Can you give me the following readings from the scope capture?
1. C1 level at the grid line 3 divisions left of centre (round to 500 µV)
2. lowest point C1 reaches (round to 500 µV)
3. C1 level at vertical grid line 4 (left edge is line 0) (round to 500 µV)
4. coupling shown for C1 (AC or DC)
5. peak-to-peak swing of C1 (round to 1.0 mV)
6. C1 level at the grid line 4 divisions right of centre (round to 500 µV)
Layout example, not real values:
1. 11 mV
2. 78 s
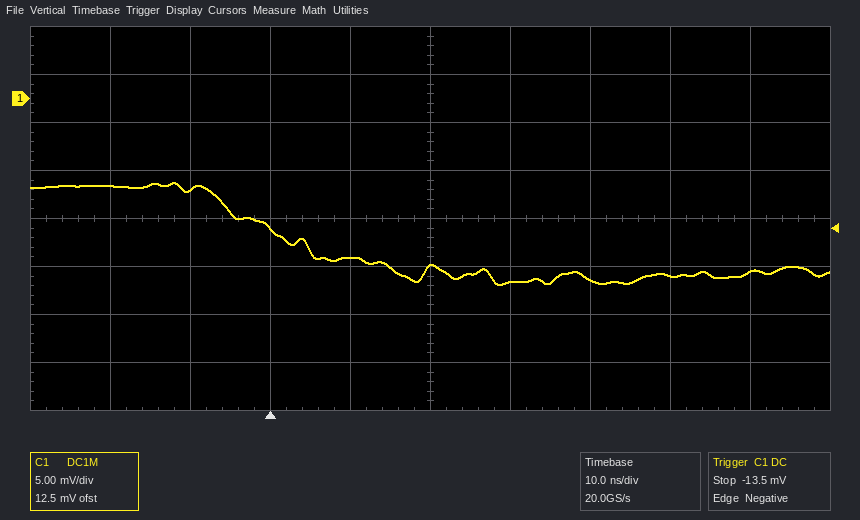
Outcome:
1. -9.5 mV
2. -19.5 mV
3. -16.5 mV
4. DC
5. 11.0 mV
6. -18.0 mV
